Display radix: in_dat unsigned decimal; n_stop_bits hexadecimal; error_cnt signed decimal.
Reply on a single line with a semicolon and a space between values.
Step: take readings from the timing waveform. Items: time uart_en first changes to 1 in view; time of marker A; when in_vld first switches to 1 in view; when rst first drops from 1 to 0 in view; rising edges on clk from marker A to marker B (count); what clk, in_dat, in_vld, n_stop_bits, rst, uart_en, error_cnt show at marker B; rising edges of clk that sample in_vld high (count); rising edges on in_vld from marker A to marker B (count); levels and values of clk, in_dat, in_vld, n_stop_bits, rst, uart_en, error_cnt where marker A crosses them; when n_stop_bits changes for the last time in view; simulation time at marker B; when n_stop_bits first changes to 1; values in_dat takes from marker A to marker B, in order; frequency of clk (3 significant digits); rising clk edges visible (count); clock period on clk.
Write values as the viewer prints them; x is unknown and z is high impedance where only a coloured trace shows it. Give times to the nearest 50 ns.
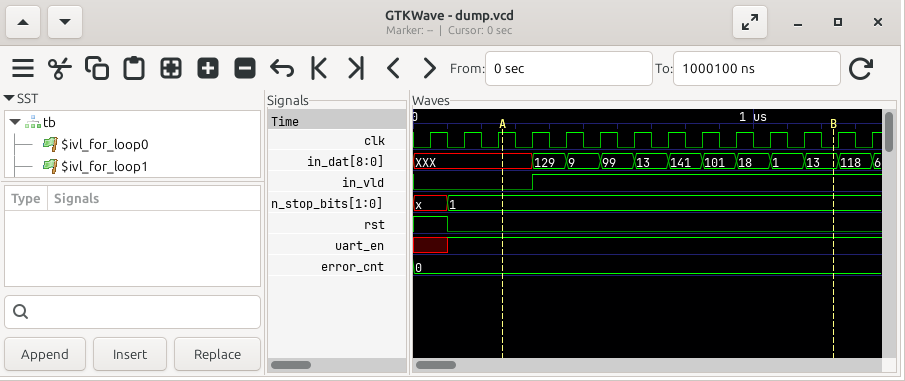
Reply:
100 ns; 250 ns; 350 ns; 100 ns; 9; clk=0, in_dat=13, in_vld=1, n_stop_bits=1, rst=0, uart_en=1, error_cnt=0; 10; 1; clk=1, in_dat=XXX, in_vld=0, n_stop_bits=1, rst=0, uart_en=1, error_cnt=0; 100 ns; 1250 ns; 100 ns; XXX, 129, 9, 99, 13, 141, 101, 18, 1, 13; 10.0 MHz; 14; 100 ns
